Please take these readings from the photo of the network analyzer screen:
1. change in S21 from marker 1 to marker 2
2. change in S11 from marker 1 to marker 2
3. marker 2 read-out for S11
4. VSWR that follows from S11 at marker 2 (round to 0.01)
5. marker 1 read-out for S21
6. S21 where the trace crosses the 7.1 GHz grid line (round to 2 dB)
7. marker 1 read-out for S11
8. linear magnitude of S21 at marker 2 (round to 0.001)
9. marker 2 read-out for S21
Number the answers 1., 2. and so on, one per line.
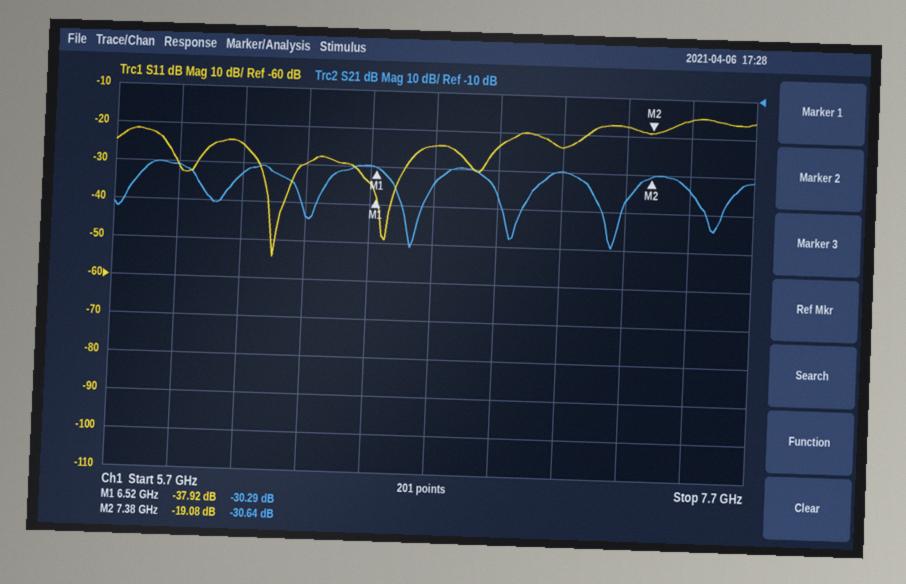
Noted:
1. -0.35 dB
2. 18.84 dB
3. -19.08 dB
4. 1.25
5. -30.29 dB
6. -30 dB
7. -37.92 dB
8. 0.029
9. -30.64 dB
